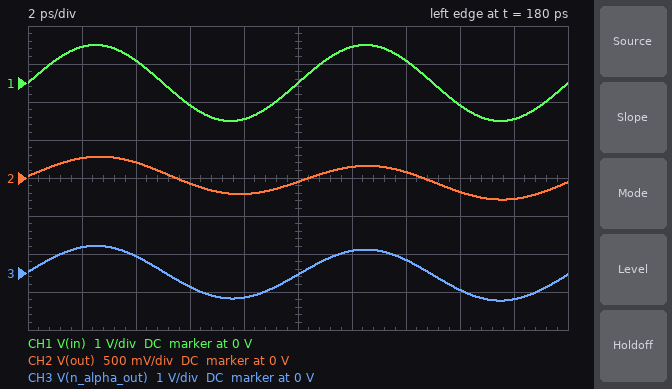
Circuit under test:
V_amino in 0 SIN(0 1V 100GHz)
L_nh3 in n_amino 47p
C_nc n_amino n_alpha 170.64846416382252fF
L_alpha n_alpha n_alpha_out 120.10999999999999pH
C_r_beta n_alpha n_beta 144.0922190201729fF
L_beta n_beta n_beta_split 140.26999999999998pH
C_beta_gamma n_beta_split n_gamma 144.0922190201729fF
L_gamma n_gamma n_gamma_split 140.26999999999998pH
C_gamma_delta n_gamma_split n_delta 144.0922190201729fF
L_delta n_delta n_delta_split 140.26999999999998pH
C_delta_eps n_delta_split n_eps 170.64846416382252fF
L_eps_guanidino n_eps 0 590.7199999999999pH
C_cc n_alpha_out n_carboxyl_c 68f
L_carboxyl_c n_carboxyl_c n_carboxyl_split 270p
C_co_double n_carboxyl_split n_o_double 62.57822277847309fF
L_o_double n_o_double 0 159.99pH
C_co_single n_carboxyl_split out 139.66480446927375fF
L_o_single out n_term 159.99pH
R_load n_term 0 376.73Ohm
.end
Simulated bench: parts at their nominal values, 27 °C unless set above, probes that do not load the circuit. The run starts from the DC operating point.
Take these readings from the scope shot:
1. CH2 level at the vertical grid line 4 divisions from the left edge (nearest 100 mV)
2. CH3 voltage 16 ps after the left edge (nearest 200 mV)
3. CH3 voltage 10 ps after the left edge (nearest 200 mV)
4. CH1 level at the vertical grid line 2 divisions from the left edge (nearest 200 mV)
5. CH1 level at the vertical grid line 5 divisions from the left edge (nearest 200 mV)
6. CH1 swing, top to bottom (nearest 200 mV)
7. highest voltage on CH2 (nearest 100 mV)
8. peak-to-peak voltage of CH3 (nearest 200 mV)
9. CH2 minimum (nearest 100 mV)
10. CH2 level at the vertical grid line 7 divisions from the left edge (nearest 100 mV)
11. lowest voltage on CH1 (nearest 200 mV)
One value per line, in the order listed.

-200 mV
-400 mV
0 V
600 mV
0 V
2.0 V
300 mV
1.4 V
-300 mV
100 mV
-1.0 V
